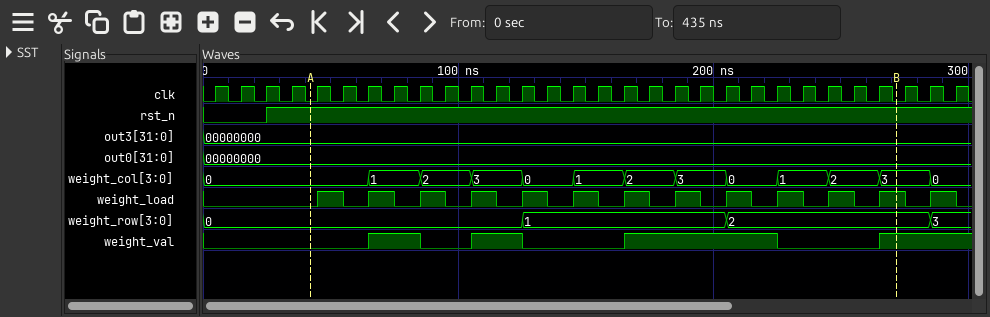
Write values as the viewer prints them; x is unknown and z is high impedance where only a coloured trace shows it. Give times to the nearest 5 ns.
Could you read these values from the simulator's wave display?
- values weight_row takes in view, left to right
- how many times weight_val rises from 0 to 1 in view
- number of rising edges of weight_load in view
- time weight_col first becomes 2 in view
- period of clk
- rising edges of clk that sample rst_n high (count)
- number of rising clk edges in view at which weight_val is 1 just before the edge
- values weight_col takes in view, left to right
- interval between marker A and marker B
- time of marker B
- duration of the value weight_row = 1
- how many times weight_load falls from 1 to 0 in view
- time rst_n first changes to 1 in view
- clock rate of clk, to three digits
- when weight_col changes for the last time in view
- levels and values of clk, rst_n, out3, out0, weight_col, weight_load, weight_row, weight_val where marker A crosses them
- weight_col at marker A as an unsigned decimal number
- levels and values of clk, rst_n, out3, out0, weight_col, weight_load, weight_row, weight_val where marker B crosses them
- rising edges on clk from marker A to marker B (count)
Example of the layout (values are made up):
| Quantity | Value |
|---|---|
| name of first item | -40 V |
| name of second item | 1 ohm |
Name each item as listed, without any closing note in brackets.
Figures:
| Quantity | Value |
|---|---|
| values weight_row takes in view, left to right | 0, 1, 2, 3 |
| how many times weight_val rises from 0 to 1 in view | 4 |
| number of rising edges of weight_load in view | 13 |
| time weight_col first becomes 2 in view | 85 ns |
| period of clk | 10 ns |
| rising edges of clk that sample rst_n high | 27 |
| number of rising clk edges in view at which weight_val is 1 just before the edge | 13 |
| values weight_col takes in view, left to right | 0, 1, 2, 3, 0, 1, 2, 3, 0, 1, 2, 3, 0 |
| interval between marker A and marker B | 230 ns |
| time of marker B | 270 ns |
| duration of the value weight_row = 1 | 80 ns |
| how many times weight_load falls from 1 to 0 in view | 13 |
| time rst_n first changes to 1 in view | 25 ns |
| clock rate of clk, to three digits | 100 MHz |
| when weight_col changes for the last time in view | 285 ns |
| levels and values of clk, rst_n, out3, out0, weight_col, weight_load, weight_row, weight_val where marker A crosses them | clk=0, rst_n=1, out3=00000000, out0=00000000, weight_col=0, weight_load=0, weight_row=0, weight_val=0 |
| weight_col at marker A as an unsigned decimal number | 0 |
| levels and values of clk, rst_n, out3, out0, weight_col, weight_load, weight_row, weight_val where marker B crosses them | clk=0, rst_n=1, out3=00000000, out0=00000000, weight_col=3, weight_load=1, weight_row=2, weight_val=1 |
| rising edges on clk from marker A to marker B | 23 |
